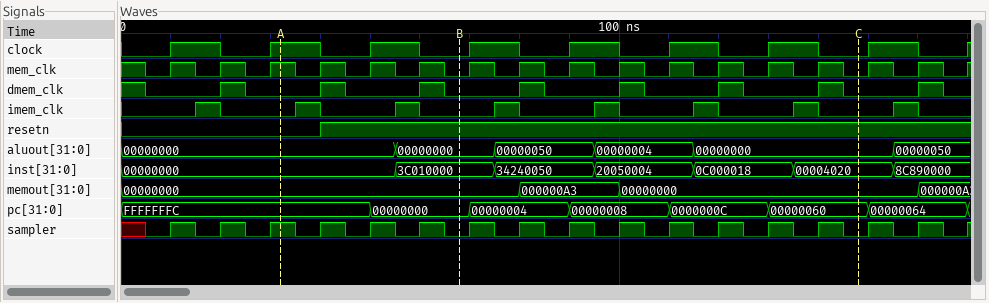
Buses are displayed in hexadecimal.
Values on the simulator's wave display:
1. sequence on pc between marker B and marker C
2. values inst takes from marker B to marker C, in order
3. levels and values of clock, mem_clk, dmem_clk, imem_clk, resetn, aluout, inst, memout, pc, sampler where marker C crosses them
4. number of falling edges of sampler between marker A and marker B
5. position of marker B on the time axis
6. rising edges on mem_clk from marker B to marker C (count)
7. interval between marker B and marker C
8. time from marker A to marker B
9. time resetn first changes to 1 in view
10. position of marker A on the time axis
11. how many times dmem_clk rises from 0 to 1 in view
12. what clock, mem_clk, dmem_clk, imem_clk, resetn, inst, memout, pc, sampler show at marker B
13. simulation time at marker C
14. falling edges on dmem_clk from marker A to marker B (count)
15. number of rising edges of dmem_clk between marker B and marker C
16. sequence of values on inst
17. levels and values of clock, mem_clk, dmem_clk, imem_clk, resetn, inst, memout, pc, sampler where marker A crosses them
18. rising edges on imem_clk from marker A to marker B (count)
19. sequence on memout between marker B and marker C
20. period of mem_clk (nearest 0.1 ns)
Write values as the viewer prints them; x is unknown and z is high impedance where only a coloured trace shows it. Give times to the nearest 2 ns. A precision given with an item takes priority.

00000000, 00000004, 00000008, 0000000C, 00000060
3C010000, 34240050, 20050004, 0C000018, 00004020
clock=0, mem_clk=0, dmem_clk=0, imem_clk=0, resetn=1, aluout=00000000, inst=00004020, memout=00000000, pc=00000060, sampler=0
4
68 ns
8
80 ns
36 ns
40 ns
32 ns
8
clock=0, mem_clk=0, dmem_clk=0, imem_clk=0, resetn=1, inst=3C010000, memout=00000000, pc=00000000, sampler=0
148 ns
2
4
00000000, 3C010000, 34240050, 20050004, 0C000018, 00004020, 8C890000
clock=1, mem_clk=1, dmem_clk=0, imem_clk=0, resetn=0, inst=00000000, memout=00000000, pc=FFFFFFFC, sampler=1
2
00000000, 000000A3, 00000000
10 ns
